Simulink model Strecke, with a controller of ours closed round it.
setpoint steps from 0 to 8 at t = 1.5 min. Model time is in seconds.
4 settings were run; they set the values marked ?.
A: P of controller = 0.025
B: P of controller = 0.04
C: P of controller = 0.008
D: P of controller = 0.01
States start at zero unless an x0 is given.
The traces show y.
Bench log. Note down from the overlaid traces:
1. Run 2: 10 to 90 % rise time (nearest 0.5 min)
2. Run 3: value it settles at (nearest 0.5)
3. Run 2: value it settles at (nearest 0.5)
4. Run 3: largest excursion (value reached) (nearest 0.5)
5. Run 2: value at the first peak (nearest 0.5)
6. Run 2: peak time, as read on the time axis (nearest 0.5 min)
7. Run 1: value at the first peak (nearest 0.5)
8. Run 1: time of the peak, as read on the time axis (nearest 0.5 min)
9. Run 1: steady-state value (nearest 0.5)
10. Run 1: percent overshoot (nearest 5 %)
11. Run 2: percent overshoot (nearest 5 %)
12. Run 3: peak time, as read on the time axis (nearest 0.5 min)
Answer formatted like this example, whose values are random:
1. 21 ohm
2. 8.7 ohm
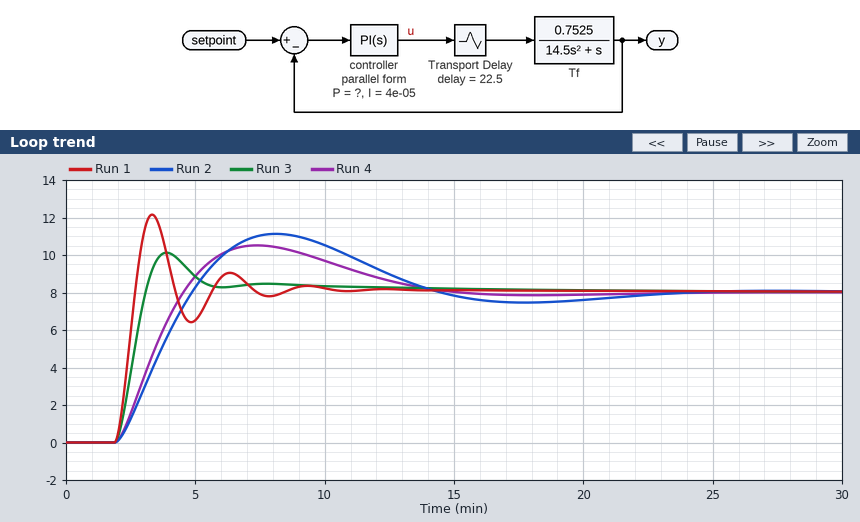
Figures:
1. 2.0 min
2. 8.0
3. 8.0
4. 10.0
5. 11.0
6. 8.0 min
7. 12.0
8. 3.5 min
9. 8.0
10. 50 %
11. 40 %
12. 4.0 min
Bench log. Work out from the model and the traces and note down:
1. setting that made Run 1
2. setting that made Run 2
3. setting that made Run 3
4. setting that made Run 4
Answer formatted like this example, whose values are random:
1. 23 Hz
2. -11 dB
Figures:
1. B
2. C
3. A
4. D
